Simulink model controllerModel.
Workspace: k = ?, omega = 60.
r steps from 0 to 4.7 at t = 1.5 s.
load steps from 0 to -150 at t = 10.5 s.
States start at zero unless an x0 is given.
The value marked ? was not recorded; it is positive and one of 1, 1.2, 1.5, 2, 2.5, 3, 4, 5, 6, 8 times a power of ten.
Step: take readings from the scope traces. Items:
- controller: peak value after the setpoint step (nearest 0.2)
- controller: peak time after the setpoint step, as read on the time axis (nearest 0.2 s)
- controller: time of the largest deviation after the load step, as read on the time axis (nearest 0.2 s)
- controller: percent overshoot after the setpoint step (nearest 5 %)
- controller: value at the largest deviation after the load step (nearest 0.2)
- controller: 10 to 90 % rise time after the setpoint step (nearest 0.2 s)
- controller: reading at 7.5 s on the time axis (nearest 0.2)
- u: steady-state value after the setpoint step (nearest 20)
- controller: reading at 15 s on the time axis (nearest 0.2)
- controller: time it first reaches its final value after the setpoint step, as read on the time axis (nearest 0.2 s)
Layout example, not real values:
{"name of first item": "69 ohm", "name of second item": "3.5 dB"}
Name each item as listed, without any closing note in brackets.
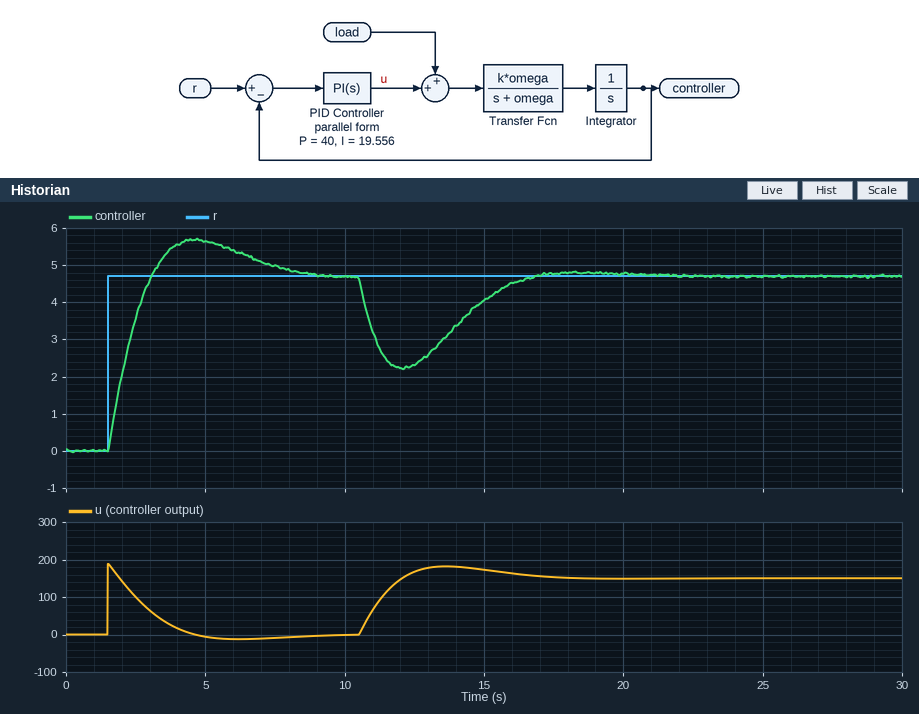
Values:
{"controller: peak value after the setpoint step": "5.6", "controller: peak time after the setpoint step, as read on the time axis": "4.6 s", "controller: time of the largest deviation after the load step, as read on the time axis": "12.0 s", "controller: percent overshoot after the setpoint step": "20 %", "controller: value at the largest deviation after the load step": "2.2", "controller: 10 to 90 % rise time after the setpoint step": "1.2 s", "controller: reading at 7.5 s on the time axis": "5.0", "u: steady-state value after the setpoint step": "0", "controller: reading at 15 s on the time axis": "4.0", "controller: time it first reaches its final value after the setpoint step, as read on the time axis": "3.0 s"}
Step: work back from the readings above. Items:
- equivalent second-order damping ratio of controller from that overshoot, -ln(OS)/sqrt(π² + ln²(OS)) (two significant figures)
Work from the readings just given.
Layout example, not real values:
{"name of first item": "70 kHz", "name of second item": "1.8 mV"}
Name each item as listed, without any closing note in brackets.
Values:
{"equivalent second-order damping ratio of controller from that overshoot, -ln(OS)/sqrt(π² + ln²(OS))": "0.46"}
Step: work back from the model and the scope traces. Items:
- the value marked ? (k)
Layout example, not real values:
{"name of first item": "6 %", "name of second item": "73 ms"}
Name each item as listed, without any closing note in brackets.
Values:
{"the value marked ?": "0.025"}
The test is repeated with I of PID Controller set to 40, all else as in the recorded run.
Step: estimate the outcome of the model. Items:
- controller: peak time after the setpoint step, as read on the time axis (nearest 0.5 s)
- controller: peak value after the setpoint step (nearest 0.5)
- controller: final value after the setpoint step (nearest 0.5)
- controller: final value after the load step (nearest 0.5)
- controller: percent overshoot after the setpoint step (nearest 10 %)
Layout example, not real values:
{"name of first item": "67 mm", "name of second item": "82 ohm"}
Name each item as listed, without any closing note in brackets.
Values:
{"controller: peak time after the setpoint step, as read on the time axis": "4.0 s", "controller: peak value after the setpoint step": "6.0", "controller: final value after the setpoint step": "4.5", "controller: final value after the load step": "4.5", "controller: percent overshoot after the setpoint step": "30 %"}
